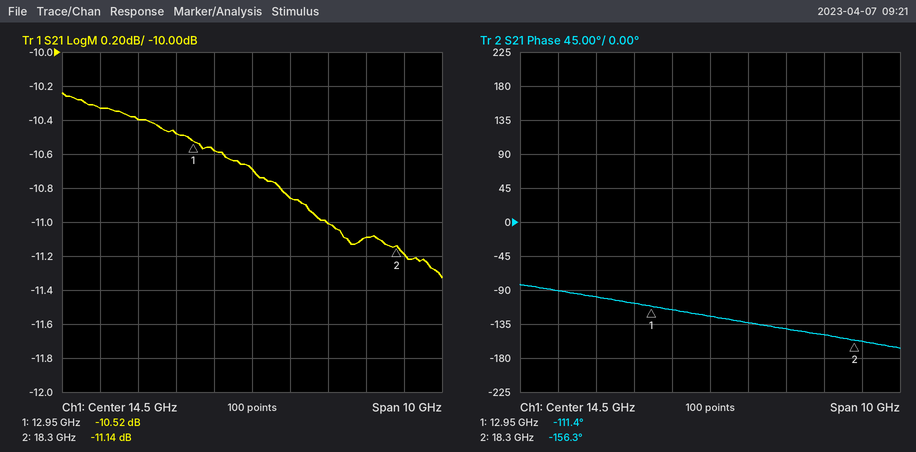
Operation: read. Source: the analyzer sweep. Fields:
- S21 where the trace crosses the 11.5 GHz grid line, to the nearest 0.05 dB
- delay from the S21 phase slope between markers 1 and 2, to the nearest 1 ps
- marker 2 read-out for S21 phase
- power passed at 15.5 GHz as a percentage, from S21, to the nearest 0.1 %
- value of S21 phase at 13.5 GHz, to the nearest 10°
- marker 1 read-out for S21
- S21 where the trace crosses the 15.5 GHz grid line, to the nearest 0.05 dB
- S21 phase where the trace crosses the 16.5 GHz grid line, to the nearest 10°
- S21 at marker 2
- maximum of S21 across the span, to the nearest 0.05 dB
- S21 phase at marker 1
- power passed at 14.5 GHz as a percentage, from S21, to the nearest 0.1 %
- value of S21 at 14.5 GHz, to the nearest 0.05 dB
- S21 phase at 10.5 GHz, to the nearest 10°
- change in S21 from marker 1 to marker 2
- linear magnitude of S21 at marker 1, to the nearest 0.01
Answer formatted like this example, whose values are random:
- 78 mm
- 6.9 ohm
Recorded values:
- -10.40 dB
- 23 ps
- -156.3°
- 8.2 %
- -120°
- -10.52 dB
- -10.85 dB
- -140°
- -11.14 dB
- -10.25 dB
- -111.4°
- 8.5 %
- -10.70 dB
- -90°
- -0.62 dB
- 0.30
